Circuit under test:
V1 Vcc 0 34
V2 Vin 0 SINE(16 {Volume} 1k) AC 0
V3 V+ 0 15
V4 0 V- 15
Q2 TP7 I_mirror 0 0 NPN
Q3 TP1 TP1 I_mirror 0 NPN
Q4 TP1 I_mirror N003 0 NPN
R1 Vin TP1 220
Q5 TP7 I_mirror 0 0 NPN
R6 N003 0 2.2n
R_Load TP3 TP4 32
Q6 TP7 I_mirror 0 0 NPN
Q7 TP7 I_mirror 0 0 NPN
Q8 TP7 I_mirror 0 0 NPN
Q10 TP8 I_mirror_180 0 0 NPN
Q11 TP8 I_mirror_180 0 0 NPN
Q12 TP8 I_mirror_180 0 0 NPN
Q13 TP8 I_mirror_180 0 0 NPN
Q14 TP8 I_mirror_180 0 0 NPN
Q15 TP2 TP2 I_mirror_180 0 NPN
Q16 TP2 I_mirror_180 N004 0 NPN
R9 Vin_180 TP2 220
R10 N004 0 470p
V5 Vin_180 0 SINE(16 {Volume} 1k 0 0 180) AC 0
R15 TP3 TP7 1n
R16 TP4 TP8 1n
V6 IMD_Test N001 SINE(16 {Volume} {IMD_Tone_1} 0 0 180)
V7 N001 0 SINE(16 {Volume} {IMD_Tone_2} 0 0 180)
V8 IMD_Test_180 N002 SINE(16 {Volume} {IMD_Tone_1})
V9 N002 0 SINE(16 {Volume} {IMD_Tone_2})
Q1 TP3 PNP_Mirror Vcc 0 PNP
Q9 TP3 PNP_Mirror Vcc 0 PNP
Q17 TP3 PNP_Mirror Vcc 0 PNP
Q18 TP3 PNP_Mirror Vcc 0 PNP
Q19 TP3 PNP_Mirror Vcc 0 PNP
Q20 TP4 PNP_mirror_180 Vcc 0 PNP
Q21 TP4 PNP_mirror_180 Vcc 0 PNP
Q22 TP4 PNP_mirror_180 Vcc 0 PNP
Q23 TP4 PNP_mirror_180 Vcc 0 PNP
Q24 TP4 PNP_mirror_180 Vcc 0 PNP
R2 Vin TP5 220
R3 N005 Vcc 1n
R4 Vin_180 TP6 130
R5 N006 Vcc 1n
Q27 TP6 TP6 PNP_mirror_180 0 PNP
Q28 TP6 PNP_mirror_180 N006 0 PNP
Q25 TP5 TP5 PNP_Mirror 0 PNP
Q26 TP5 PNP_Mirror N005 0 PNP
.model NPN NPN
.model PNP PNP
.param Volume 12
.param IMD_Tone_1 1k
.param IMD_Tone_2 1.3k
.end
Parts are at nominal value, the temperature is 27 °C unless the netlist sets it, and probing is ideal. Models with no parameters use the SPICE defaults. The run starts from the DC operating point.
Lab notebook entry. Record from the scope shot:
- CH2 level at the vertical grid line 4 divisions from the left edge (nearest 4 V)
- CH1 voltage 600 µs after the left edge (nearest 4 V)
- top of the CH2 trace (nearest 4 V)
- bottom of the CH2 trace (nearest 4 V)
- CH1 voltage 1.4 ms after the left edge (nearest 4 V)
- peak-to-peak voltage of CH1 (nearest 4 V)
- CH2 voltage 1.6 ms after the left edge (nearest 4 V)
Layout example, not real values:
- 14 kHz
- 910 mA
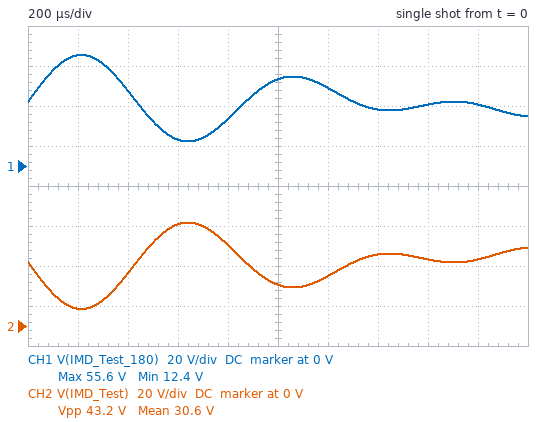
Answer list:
- 40 V
- 12 V
- 52 V
- 8 V
- 28 V
- 44 V
- 32 V
